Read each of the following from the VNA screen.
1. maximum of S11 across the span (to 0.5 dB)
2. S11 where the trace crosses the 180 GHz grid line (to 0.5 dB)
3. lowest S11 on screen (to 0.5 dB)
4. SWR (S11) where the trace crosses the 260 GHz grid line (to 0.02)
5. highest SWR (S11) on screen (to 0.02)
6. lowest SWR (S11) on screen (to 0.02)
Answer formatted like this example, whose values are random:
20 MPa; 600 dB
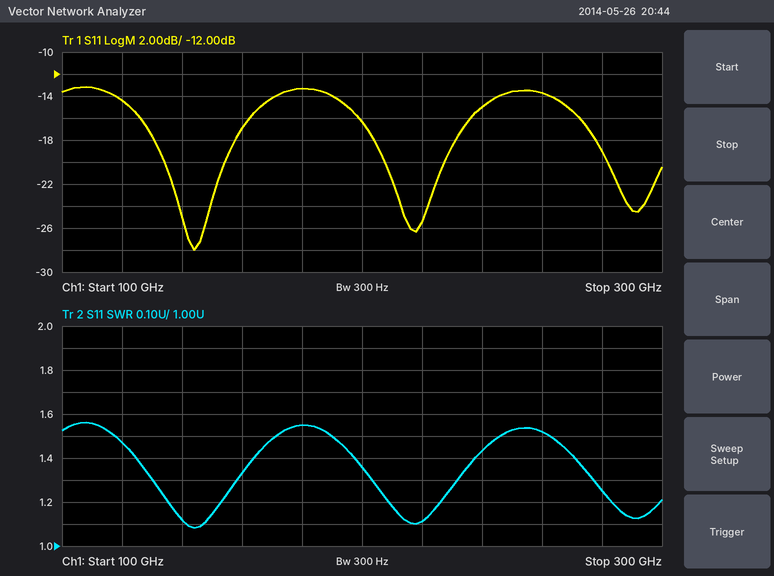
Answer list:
-13.0 dB; -13.5 dB; -28.0 dB; 1.52; 1.56; 1.08
